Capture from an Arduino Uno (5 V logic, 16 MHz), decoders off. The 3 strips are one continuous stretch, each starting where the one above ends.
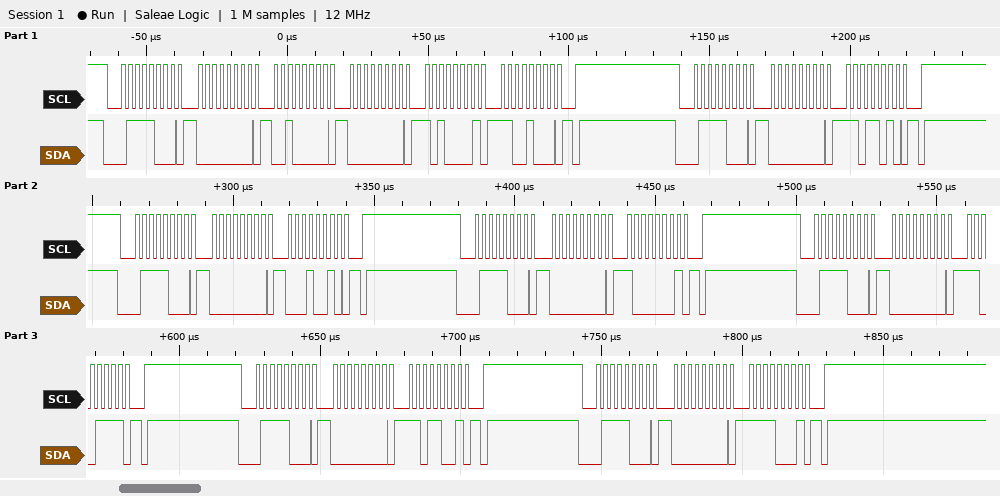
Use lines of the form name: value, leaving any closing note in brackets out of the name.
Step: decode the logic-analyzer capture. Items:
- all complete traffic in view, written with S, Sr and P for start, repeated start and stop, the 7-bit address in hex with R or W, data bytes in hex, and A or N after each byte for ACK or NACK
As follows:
all complete traffic in view, written with S, Sr and P for start, repeated start and stop, the 7-bit address in hex with R or W, data bytes in hex, and A or N after each byte for ACK or NACK: S 3CW A 00 A 20 A 00 A A1 A C8 A P S 3CW A 00 A DA A P S 3CW A 00 A 12 A P S 3CW A 00 A 81 A P S 3CW A 00 A CF A P S 3CW A 00 A D9 A P S 3CW A 00 A F1 A P
